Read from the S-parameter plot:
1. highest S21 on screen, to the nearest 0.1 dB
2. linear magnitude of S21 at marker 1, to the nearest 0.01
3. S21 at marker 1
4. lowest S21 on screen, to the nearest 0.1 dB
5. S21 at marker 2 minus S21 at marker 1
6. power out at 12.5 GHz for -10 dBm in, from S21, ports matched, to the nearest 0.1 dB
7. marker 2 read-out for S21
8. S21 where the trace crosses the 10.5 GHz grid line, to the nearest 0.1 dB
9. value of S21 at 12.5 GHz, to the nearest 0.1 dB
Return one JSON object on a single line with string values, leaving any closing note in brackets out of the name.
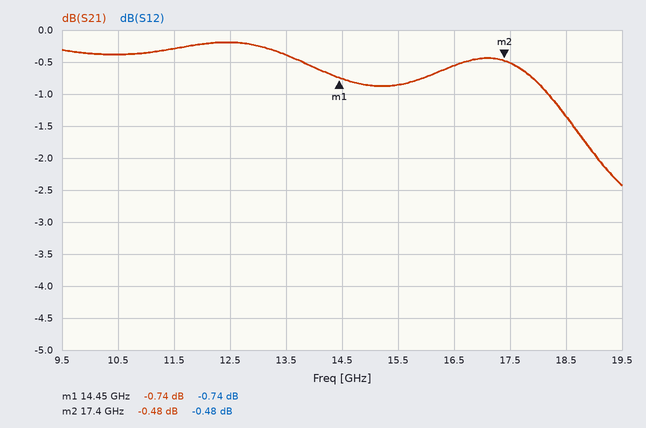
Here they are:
{"highest S21 on screen, to the nearest 0.1 dB": "-0.2 dB", "linear magnitude of S21 at marker 1, to the nearest 0.01": "0.92", "S21 at marker 1": "-0.74 dB", "lowest S21 on screen, to the nearest 0.1 dB": "-2.4 dB", "S21 at marker 2 minus S21 at marker 1": "0.26 dB", "power out at 12.5 GHz for -10 dBm in, from S21, ports matched, to the nearest 0.1 dB": "-10.2 dBm", "marker 2 read-out for S21": "-0.48 dB", "S21 where the trace crosses the 10.5 GHz grid line, to the nearest 0.1 dB": "-0.4 dB", "value of S21 at 12.5 GHz, to the nearest 0.1 dB": "-0.2 dB"}
